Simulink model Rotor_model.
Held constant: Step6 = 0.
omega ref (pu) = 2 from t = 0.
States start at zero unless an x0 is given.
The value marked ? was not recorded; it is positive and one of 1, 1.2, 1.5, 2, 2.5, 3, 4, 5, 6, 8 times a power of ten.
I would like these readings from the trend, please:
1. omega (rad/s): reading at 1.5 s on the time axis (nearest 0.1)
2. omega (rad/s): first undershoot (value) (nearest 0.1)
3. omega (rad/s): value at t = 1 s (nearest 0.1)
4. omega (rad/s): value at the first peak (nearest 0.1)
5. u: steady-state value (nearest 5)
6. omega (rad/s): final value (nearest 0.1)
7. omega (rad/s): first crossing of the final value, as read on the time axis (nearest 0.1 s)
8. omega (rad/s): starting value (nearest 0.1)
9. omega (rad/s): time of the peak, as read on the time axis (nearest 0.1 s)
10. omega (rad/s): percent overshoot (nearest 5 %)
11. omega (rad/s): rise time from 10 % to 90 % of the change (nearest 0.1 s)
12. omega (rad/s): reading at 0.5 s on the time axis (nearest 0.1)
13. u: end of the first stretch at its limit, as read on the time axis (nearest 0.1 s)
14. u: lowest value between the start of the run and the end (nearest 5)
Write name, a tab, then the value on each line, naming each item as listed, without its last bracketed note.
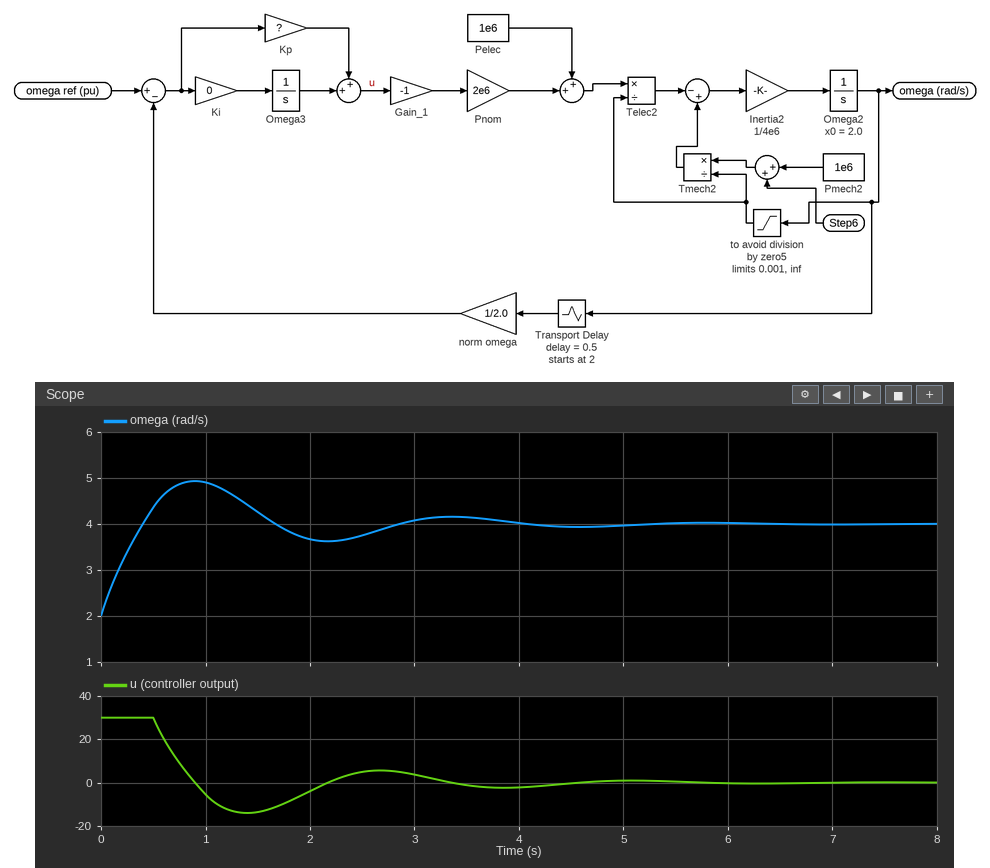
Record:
omega (rad/s): reading at 1.5 s on the time axis	4.3
omega (rad/s): first undershoot (value)	3.6
omega (rad/s): value at t = 1 s	4.9
omega (rad/s): value at the first peak	4.9
u: steady-state value	0
omega (rad/s): final value	4.0
omega (rad/s): first crossing of the final value, as read on the time axis	0.4 s
omega (rad/s): starting value	2.0
omega (rad/s): time of the peak, as read on the time axis	0.9 s
omega (rad/s): percent overshoot	45 %
omega (rad/s): rise time from 10 % to 90 % of the change	0.3 s
omega (rad/s): reading at 0.5 s on the time axis	4.4
u: end of the first stretch at its limit, as read on the time axis	0.5 s
u: lowest value between the start of the run and the end	-15
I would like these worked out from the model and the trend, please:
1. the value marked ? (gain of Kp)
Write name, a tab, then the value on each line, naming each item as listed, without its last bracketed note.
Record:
the value marked ?	30
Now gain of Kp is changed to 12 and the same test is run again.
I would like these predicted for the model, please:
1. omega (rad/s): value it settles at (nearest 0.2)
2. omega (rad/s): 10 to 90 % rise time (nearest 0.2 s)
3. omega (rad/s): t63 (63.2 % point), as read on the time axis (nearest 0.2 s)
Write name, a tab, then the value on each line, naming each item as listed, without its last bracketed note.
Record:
omega (rad/s): value it settles at	4.0
omega (rad/s): 10 to 90 % rise time	1.0 s
omega (rad/s): t63 (63.2 % point), as read on the time axis	0.6 s
